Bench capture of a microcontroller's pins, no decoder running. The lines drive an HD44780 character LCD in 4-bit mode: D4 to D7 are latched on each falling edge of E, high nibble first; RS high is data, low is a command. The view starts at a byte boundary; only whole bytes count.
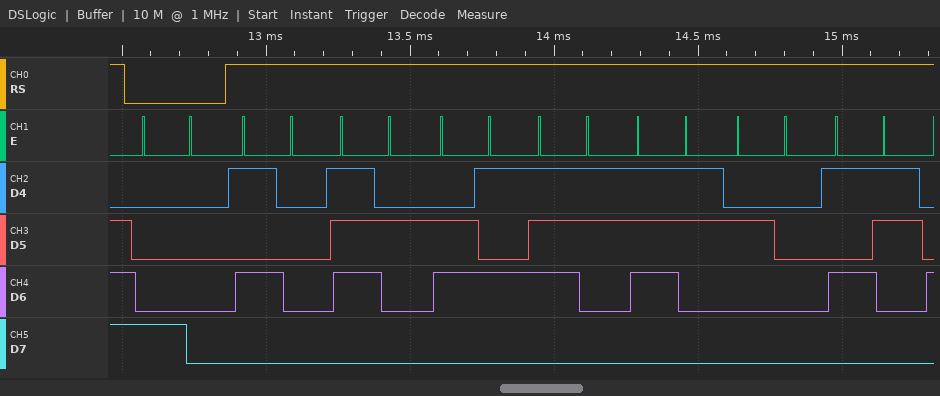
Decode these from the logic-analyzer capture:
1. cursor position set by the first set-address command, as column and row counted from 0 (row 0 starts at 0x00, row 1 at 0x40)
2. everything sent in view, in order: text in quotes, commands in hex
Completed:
column 0, row 0
0x80 "Press S"
